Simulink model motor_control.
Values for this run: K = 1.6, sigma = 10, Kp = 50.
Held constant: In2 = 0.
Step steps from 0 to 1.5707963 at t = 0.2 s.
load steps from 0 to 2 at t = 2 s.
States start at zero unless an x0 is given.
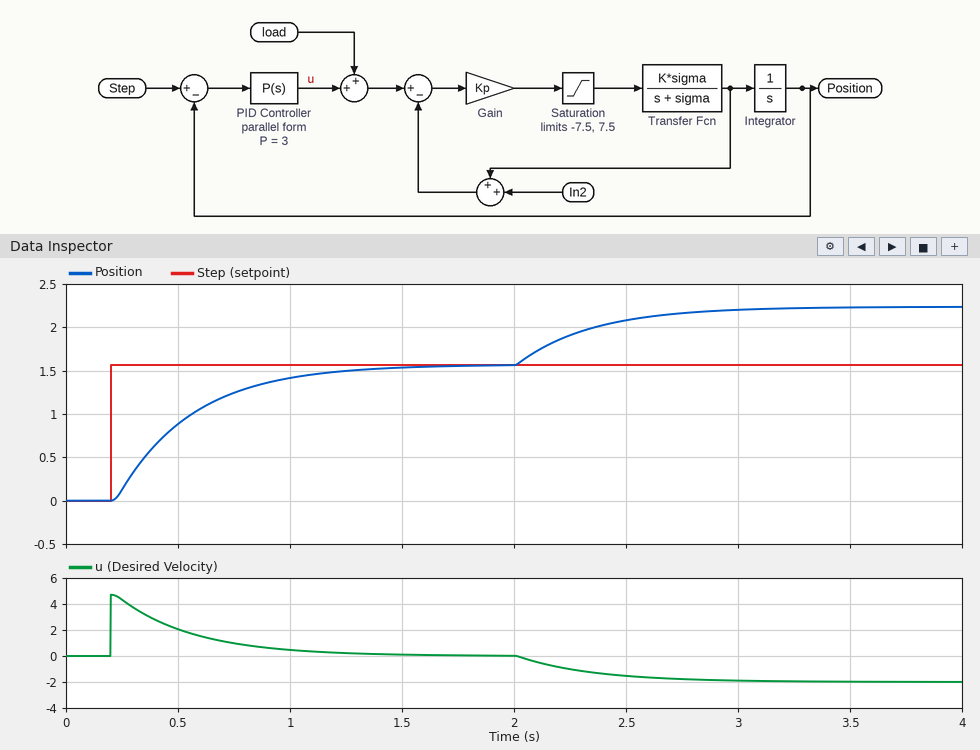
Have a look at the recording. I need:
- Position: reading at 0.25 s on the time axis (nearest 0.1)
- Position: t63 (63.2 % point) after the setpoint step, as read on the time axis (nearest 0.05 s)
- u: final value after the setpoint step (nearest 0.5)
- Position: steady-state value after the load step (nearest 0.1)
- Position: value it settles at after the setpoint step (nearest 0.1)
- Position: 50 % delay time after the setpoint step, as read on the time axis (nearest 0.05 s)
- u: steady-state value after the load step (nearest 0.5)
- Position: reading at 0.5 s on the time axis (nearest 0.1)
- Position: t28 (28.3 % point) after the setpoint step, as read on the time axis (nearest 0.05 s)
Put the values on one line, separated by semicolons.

0.1; 0.55 s; 0.0; 2.2; 1.6; 0.45 s; -2.0; 0.9; 0.35 s
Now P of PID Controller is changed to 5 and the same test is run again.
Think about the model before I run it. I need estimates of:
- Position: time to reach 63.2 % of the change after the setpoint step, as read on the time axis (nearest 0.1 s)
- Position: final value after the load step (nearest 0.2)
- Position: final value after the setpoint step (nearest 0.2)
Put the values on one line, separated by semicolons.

0.4 s; 2.0; 1.6
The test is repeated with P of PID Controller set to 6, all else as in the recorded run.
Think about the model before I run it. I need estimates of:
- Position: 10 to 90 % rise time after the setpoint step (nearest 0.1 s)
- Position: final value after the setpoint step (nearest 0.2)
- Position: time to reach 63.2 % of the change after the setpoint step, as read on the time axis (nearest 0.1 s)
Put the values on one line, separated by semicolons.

0.4 s; 1.6; 0.4 s
